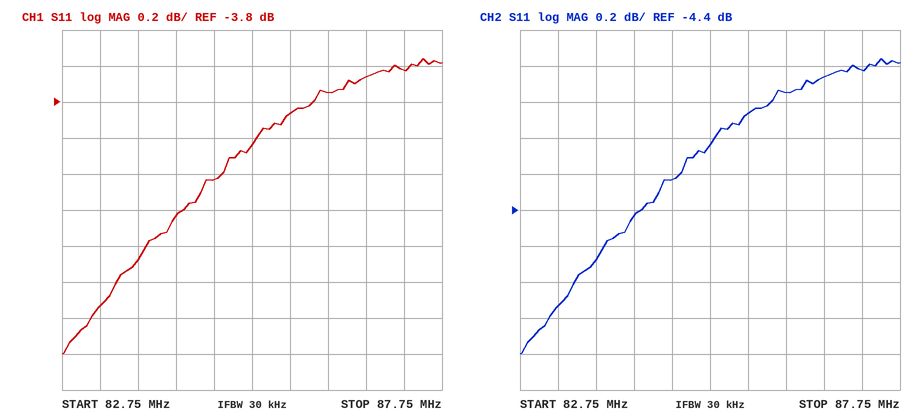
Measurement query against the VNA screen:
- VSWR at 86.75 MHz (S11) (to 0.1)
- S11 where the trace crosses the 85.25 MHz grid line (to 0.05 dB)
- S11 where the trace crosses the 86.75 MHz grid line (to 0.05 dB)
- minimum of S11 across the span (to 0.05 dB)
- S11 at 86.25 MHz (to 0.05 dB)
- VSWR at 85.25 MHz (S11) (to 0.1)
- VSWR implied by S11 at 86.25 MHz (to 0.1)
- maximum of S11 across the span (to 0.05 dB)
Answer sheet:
4.8
-4.05 dB
-3.65 dB
-5.20 dB
-3.75 dB
4.4
4.7
-3.55 dB
